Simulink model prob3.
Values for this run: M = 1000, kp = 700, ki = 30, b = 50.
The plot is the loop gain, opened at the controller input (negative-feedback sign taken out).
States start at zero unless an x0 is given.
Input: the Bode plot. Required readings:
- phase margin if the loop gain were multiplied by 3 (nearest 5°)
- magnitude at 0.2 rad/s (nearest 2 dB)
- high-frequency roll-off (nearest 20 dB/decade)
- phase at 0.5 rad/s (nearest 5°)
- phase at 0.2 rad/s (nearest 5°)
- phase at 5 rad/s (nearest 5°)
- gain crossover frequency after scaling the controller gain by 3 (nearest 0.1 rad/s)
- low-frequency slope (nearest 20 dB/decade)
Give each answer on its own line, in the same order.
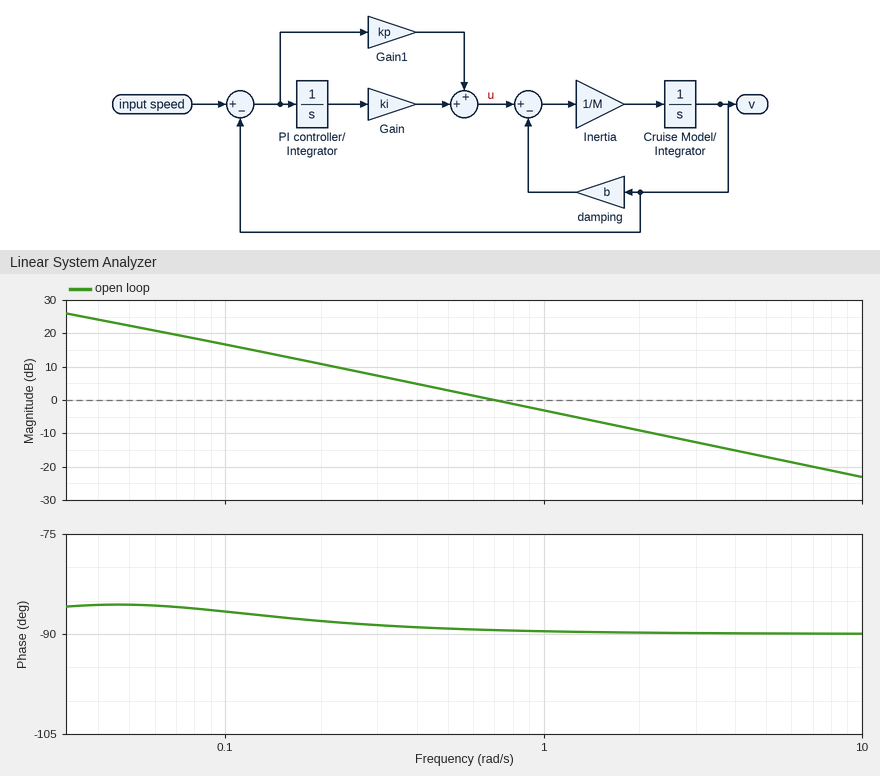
90°
10 dB
-20 dB/decade
-90°
-90°
-90°
2.1 rad/s
-20 dB/decade
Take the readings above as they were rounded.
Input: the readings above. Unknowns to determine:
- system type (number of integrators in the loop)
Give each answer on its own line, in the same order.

1
